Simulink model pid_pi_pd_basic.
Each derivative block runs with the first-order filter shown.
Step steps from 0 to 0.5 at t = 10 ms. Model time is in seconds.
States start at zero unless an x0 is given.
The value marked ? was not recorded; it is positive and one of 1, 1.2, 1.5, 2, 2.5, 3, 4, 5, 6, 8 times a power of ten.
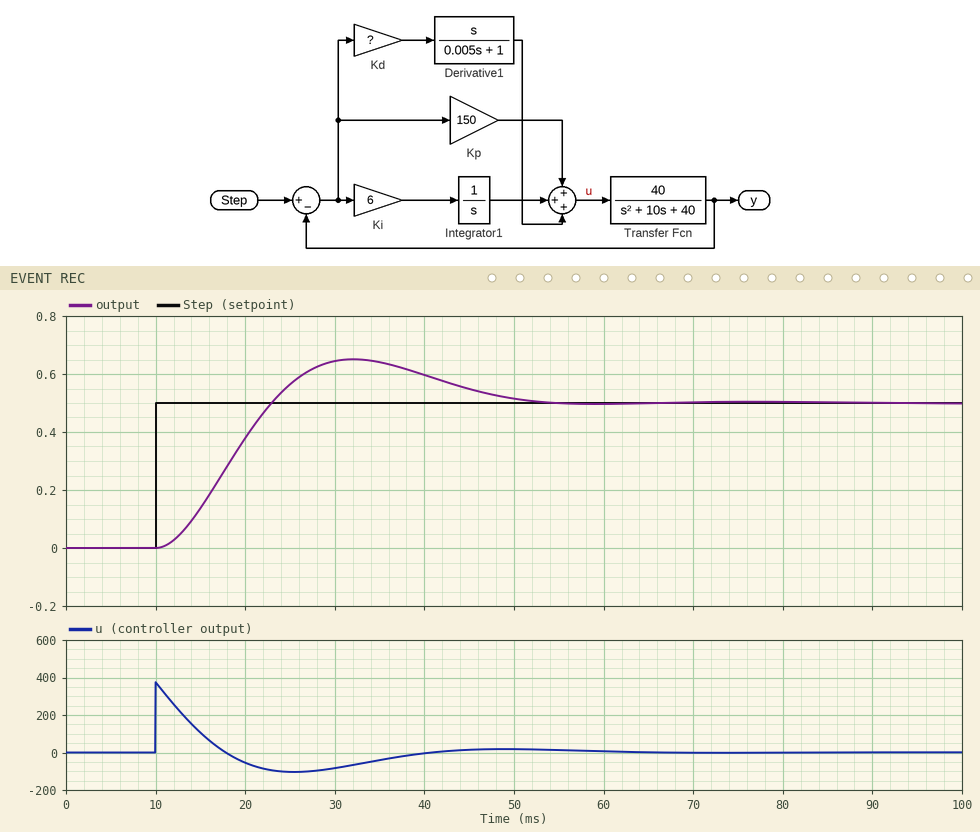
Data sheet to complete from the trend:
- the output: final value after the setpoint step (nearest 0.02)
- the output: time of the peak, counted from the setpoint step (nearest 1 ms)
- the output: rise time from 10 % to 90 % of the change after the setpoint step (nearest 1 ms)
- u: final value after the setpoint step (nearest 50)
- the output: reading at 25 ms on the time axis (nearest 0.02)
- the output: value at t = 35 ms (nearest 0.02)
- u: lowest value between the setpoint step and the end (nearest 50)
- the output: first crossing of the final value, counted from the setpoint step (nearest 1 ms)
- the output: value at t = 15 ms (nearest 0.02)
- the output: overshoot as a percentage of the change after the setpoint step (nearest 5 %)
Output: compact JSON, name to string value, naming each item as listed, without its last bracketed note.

{"the output: final value after the setpoint step": "0.50", "the output: time of the peak, counted from the setpoint step": "22 ms", "the output: rise time from 10 % to 90 % of the change after the setpoint step": "9 ms", "u: final value after the setpoint step": "0", "the output: reading at 25 ms on the time axis": "0.56", "the output: value at t = 35 ms": "0.64", "u: lowest value between the setpoint step and the end": "-100", "the output: first crossing of the final value, counted from the setpoint step": "13 ms", "the output: value at t = 15 ms": "0.14", "the output: overshoot as a percentage of the change after the setpoint step": "30 %"}
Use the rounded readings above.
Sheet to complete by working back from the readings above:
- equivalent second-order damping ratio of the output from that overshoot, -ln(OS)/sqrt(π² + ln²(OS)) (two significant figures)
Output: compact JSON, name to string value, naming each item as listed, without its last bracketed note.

{"equivalent second-order damping ratio of the output from that overshoot, -ln(OS)/sqrt(π² + ln²(OS))": "0.36"}
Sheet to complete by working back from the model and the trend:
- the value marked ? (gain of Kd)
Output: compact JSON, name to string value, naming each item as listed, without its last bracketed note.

{"the value marked ?": "3"}
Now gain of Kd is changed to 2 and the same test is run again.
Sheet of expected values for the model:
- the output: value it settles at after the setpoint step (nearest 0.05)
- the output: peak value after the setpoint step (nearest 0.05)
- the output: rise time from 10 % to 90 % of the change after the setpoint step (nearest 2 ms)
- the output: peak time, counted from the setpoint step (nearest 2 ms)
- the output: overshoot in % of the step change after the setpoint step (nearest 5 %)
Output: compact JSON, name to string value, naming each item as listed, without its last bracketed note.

{"the output: value it settles at after the setpoint step": "0.50", "the output: peak value after the setpoint step": "0.70", "the output: rise time from 10 % to 90 % of the change after the setpoint step": "10 ms", "the output: peak time, counted from the setpoint step": "26 ms", "the output: overshoot in % of the step change after the setpoint step": "35 %"}
